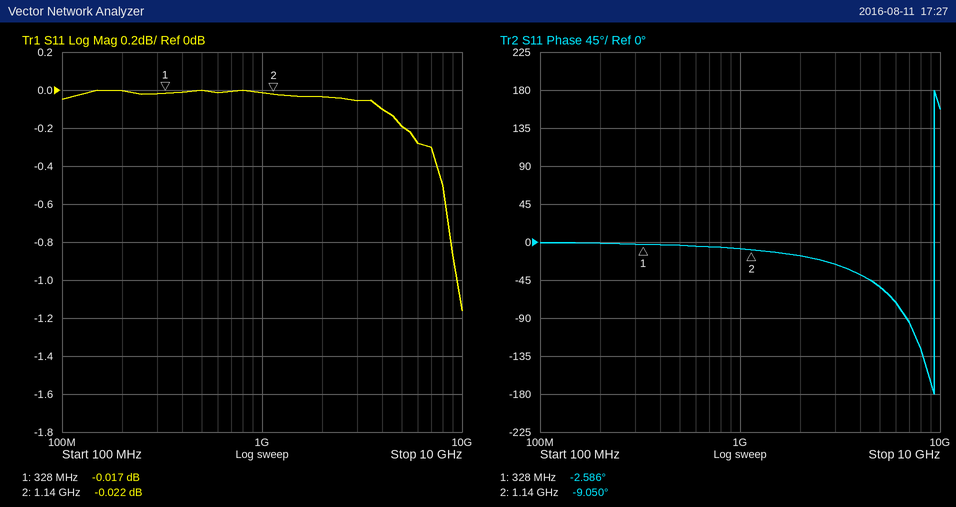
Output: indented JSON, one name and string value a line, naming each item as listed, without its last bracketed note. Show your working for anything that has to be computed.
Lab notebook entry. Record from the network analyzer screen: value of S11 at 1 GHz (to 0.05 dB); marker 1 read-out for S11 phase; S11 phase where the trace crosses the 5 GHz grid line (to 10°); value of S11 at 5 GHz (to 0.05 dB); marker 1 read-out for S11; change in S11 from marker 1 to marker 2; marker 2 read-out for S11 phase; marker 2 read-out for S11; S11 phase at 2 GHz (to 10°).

{
  "value of S11 at 1 GHz": "0.00 dB",
  "marker 1 read-out for S11 phase": "-2.586°",
  "S11 phase where the trace crosses the 5 GHz grid line": "-50°",
  "value of S11 at 5 GHz": "-0.20 dB",
  "marker 1 read-out for S11": "-0.017 dB",
  "change in S11 from marker 1 to marker 2": "-0.022 − (-0.017) = -0.005 dB",
  "marker 2 read-out for S11 phase": "-9.050°",
  "marker 2 read-out for S11": "-0.022 dB",
  "S11 phase at 2 GHz": "-20°"
}
